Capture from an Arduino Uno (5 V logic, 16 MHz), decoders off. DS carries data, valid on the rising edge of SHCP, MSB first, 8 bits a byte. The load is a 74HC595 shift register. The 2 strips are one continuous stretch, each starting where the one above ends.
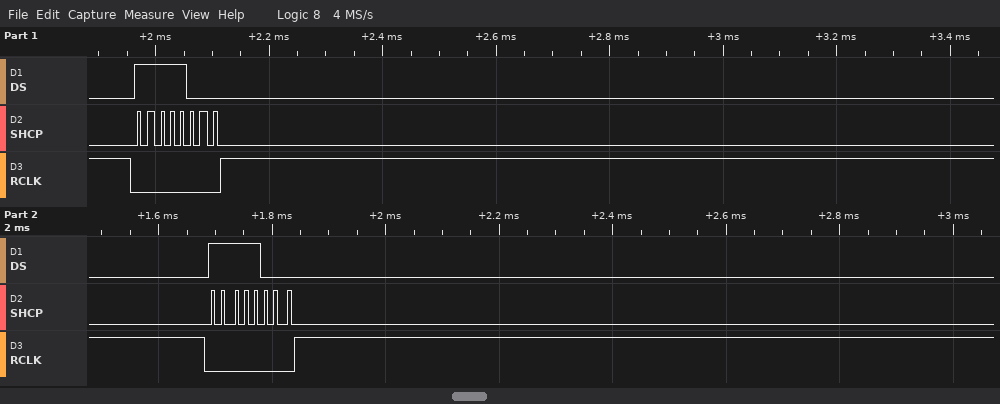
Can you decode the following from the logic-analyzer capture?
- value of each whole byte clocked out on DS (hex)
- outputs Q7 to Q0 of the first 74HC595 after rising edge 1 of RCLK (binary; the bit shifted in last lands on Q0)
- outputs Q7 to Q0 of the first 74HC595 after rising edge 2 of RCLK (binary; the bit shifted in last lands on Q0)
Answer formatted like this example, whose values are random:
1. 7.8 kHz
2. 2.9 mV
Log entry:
1. 0xF8 0xF8
2. 11111000
3. 11111000
